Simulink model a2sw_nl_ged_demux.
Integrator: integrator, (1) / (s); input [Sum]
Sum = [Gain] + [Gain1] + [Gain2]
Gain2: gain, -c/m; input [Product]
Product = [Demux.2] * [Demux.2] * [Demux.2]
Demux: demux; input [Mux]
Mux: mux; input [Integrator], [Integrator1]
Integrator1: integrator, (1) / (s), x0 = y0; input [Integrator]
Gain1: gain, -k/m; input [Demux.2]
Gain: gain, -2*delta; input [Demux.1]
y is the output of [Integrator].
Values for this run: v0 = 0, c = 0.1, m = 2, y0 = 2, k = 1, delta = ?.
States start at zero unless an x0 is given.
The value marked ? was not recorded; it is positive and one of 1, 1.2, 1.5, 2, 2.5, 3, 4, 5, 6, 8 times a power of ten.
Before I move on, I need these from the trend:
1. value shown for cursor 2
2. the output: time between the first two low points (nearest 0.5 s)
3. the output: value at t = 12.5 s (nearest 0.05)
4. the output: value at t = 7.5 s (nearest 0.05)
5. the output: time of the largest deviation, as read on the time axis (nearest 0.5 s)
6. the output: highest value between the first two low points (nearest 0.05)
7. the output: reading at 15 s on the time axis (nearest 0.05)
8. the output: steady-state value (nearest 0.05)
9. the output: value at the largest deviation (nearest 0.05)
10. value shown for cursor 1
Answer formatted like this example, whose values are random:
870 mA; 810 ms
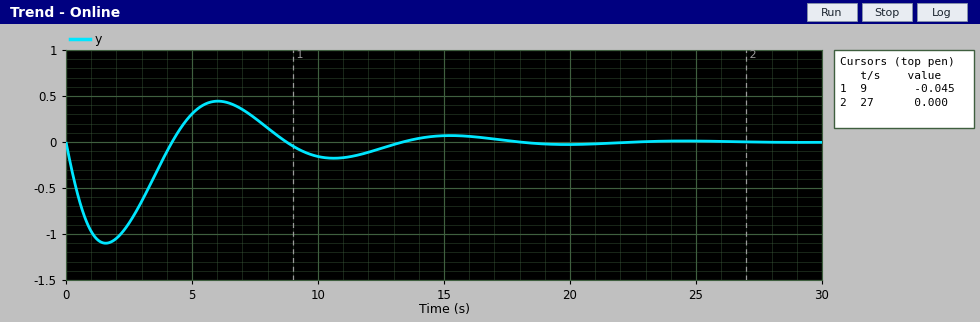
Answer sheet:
0.000; 9.0 s; -0.05; 0.25; 1.5 s; 0.45; 0.05; 0.00; -1.10; -0.045
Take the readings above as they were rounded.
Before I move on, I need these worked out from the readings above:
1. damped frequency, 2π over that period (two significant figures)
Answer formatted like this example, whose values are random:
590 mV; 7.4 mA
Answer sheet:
0.70 rad/s
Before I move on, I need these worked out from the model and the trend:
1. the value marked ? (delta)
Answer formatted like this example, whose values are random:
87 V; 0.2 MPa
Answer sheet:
0.2
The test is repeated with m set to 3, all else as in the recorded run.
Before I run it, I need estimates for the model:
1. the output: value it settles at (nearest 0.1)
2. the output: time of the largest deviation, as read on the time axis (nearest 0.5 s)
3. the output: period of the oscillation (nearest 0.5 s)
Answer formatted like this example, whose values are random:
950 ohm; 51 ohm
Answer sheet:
0.0; 2.0 s; 11.5 s
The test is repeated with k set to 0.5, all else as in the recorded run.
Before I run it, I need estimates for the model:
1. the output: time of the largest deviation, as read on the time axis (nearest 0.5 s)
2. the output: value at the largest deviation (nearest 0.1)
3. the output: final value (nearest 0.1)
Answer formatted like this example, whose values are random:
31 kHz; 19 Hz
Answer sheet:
2.0 s; -0.8; 0.0
